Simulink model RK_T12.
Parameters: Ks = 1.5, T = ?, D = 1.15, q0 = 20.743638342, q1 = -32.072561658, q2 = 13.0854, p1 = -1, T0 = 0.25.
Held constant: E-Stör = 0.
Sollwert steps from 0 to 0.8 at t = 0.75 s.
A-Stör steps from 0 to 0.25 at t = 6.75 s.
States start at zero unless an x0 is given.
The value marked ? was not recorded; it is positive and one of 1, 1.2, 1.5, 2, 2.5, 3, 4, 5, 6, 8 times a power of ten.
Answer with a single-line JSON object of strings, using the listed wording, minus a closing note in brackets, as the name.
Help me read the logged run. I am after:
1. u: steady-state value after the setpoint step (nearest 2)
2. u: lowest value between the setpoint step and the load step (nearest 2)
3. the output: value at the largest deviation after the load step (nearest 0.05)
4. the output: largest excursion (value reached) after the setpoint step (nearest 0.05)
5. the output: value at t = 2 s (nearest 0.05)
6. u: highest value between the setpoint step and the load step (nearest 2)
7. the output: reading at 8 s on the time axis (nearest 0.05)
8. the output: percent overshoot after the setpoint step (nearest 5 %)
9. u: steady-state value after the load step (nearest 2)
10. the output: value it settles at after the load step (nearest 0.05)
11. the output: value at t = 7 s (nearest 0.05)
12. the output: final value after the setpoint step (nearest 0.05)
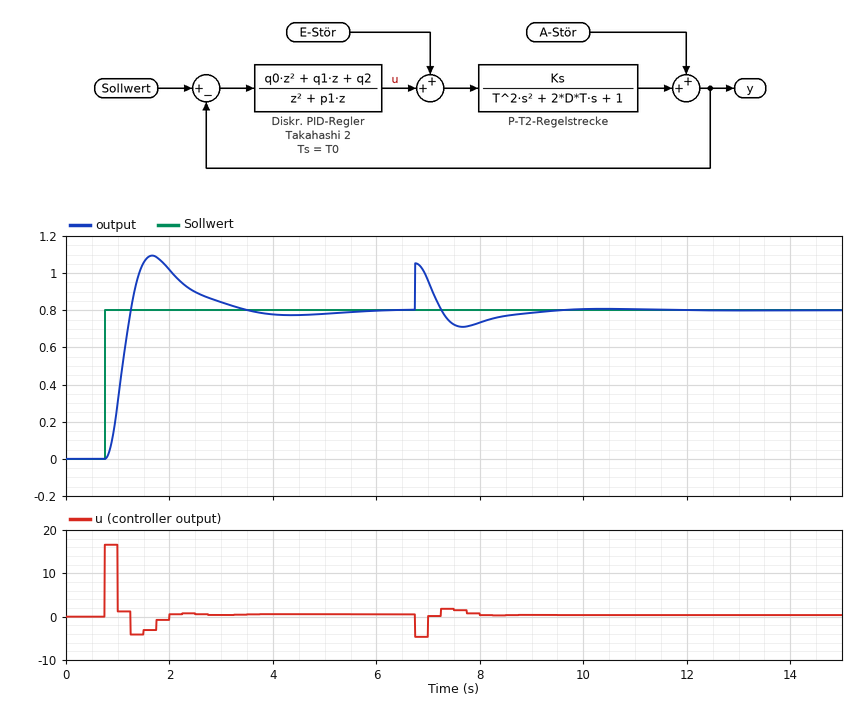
{"u: steady-state value after the setpoint step": "0", "u: lowest value between the setpoint step and the load step": "-4", "the output: value at the largest deviation after the load step": "1.05", "the output: largest excursion (value reached) after the setpoint step": "1.10", "the output: value at t = 2 s": "1.00", "u: highest value between the setpoint step and the load step": "16", "the output: reading at 8 s on the time axis": "0.75", "the output: percent overshoot after the setpoint step": "35 %", "u: steady-state value after the load step": "0", "the output: value it settles at after the load step": "0.80", "the output: value at t = 7 s": "0.95", "the output: final value after the setpoint step": "0.80"}
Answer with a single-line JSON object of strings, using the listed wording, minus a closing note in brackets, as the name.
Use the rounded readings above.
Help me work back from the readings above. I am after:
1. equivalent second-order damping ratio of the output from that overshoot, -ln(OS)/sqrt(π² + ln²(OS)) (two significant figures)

{"equivalent second-order damping ratio of the output from that overshoot, -ln(OS)/sqrt(π² + ln²(OS))": "0.32"}
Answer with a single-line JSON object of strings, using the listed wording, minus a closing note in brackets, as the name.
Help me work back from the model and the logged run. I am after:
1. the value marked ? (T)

{"the value marked ?": "1.5"}
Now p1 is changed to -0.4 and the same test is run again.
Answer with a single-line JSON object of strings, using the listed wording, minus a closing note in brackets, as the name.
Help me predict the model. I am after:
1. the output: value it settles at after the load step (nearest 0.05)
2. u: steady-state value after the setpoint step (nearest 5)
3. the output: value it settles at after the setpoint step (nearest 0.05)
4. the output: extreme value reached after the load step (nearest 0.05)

{"the output: value it settles at after the load step": "0.70", "u: steady-state value after the setpoint step": "0", "the output: value it settles at after the setpoint step": "0.65", "the output: extreme value reached after the load step": "0.90"}
